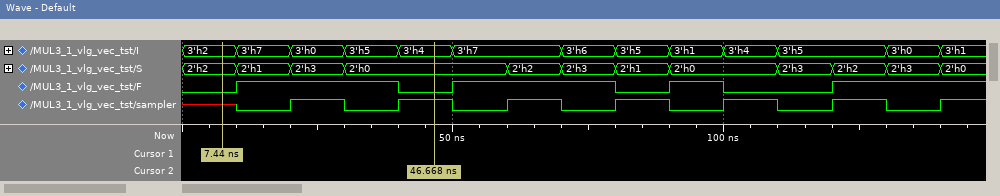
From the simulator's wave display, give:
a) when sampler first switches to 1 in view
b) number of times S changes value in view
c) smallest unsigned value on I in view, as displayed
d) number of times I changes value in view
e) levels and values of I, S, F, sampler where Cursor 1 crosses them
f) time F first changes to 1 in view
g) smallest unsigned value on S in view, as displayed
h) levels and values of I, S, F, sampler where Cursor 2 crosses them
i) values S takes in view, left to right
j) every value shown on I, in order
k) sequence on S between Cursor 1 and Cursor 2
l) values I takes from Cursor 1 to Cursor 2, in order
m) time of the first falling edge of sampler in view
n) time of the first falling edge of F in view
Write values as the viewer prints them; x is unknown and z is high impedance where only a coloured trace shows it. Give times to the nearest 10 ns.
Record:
20 ns
11
3'h0
12
I=3'h2, S=2'h2, F=0, sampler=x
10 ns
2'h0
I=3'h4, S=2'h0, F=0, sampler=1
2'h2, 2'h1, 2'h3, 2'h0, 2'h2, 2'h3, 2'h1, 2'h0, 2'h3, 2'h2, 2'h3, 2'h0
3'h2, 3'h7, 3'h0, 3'h5, 3'h4, 3'h7, 3'h6, 3'h5, 3'h1, 3'h4, 3'h5, 3'h0, 3'h1
2'h2, 2'h1, 2'h3, 2'h0
3'h2, 3'h7, 3'h0, 3'h5, 3'h4
30 ns
40 ns
